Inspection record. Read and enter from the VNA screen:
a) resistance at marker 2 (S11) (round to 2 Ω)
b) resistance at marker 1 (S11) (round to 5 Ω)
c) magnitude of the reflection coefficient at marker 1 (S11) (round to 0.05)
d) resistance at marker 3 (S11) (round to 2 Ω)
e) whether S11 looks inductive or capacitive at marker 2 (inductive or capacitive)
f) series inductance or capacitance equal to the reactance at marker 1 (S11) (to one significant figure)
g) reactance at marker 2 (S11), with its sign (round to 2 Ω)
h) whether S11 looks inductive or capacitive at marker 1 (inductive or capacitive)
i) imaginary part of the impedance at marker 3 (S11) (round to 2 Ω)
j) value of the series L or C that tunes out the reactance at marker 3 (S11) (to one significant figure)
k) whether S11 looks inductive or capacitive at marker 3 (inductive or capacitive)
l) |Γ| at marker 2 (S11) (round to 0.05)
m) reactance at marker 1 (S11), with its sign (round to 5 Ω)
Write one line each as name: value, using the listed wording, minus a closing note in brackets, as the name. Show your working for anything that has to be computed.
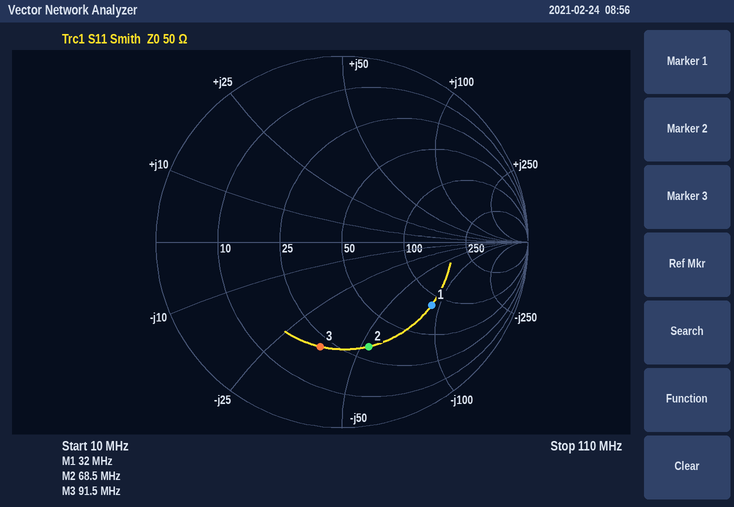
resistance at marker 2 (S11): 32 Ω
resistance at marker 1 (S11): 85 Ω
magnitude of the reflection coefficient at marker 1 (S11): 0.60
resistance at marker 3 (S11): 22 Ω
whether S11 looks inductive or capacitive at marker 2: capacitive
series inductance or capacitance equal to the reactance at marker 1 (S11): C = 1/(2π × 32 MHz × 90 Ω) ≈ 55.3 pF, so 60 pF to one significant figure
reactance at marker 2 (S11), with its sign: -54 Ω
whether S11 looks inductive or capacitive at marker 1: capacitive
imaginary part of the impedance at marker 3 (S11): -36 Ω
value of the series L or C that tunes out the reactance at marker 3 (S11): L = 36 Ω/(2π × 91.5 MHz) ≈ 62.6 nH, so 60 nH to one significant figure
whether S11 looks inductive or capacitive at marker 3: capacitive
|Γ| at marker 2 (S11): 0.60
reactance at marker 1 (S11), with its sign: -90 Ω
